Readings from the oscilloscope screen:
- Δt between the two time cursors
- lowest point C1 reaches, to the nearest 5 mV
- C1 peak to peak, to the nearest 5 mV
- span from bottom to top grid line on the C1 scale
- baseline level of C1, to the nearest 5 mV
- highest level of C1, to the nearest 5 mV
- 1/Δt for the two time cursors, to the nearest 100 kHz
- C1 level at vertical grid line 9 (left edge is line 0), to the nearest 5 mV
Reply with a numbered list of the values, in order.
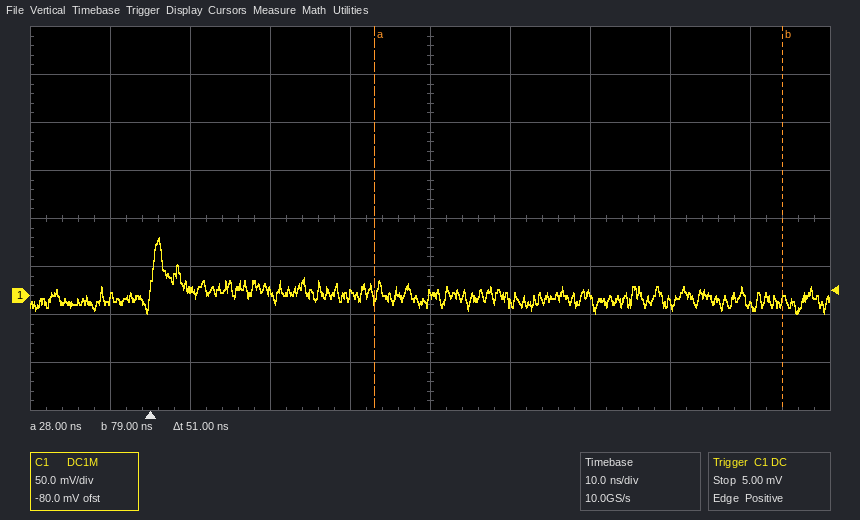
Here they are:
1. 51 ns
2. -20 mV
3. 80 mV
4. 400 mV
5. 0 mV
6. 60 mV
7. 19.6 MHz
8. -10 mV
